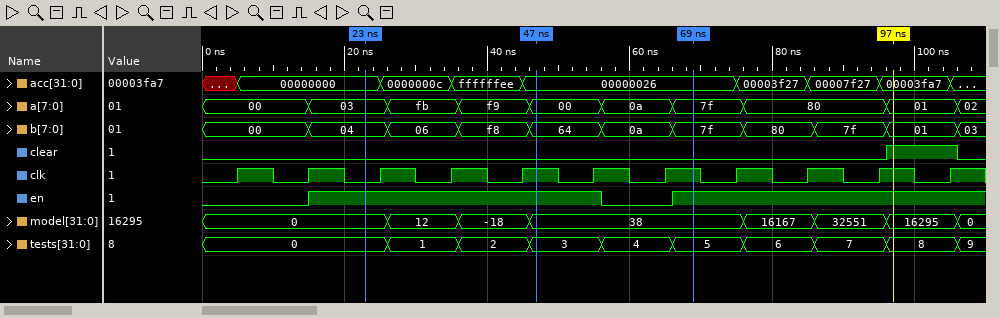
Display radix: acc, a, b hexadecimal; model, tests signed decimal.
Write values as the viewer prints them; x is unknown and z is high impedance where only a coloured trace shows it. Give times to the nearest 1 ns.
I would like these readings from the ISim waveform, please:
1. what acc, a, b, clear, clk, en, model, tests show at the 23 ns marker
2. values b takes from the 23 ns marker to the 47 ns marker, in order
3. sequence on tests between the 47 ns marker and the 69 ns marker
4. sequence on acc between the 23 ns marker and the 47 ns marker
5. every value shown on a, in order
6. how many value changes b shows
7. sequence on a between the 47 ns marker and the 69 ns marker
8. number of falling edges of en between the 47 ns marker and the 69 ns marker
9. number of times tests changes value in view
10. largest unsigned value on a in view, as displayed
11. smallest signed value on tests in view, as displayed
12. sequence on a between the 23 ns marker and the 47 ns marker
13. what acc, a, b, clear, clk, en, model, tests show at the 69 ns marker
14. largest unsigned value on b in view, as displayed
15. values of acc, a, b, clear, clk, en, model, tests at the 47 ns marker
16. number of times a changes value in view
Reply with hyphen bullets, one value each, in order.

- acc=00000000, a=03, b=04, clear=0, clk=0, en=1, model=0, tests=0
- 04, 06, f8, 64
- 3, 4, 5
- 00000000, 0000000c, ffffffee, 00000026
- 00, 03, fb, f9, 00, 0a, 7f, 80, 01, 02
- 10
- 00, 0a, 7f
- 1
- 9
- fb
- 0
- 03, fb, f9, 00
- acc=00000026, a=7f, b=7f, clear=0, clk=1, en=1, model=38, tests=5
- f8
- acc=00000026, a=00, b=64, clear=0, clk=1, en=1, model=38, tests=3
- 9
